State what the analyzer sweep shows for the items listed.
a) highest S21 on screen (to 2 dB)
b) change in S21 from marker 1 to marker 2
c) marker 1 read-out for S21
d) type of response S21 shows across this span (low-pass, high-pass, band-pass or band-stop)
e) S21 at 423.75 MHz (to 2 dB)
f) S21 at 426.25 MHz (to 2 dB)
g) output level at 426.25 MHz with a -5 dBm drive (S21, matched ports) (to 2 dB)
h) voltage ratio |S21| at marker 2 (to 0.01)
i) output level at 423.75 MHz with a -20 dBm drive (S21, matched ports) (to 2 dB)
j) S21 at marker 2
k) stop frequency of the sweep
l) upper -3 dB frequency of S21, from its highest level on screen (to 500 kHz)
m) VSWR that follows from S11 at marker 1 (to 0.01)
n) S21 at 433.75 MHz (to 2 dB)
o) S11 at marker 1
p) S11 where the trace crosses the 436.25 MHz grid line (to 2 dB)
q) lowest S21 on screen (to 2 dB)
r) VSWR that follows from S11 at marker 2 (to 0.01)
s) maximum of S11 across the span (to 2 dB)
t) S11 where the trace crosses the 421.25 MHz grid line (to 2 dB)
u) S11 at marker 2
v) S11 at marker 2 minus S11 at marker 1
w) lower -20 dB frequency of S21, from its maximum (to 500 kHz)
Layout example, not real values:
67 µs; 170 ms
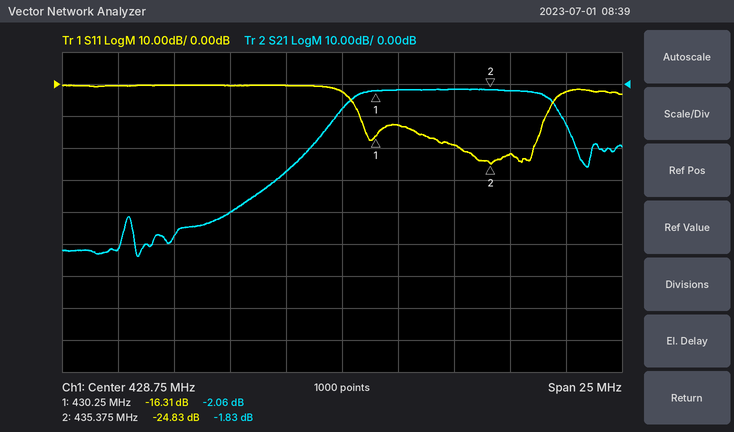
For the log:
-2 dB; 0.23 dB; -2.06 dB; band-pass; -40 dB; -28 dB; -32 dBm; 0.81; -60 dBm; -1.83 dB; 441.25 MHz; 438.0 MHz; 1.36; -2 dB; -16.31 dB; -22 dB; -54 dB; 1.12; 0 dB; 0 dB; -24.83 dB; -8.52 dB; 427.0 MHz
